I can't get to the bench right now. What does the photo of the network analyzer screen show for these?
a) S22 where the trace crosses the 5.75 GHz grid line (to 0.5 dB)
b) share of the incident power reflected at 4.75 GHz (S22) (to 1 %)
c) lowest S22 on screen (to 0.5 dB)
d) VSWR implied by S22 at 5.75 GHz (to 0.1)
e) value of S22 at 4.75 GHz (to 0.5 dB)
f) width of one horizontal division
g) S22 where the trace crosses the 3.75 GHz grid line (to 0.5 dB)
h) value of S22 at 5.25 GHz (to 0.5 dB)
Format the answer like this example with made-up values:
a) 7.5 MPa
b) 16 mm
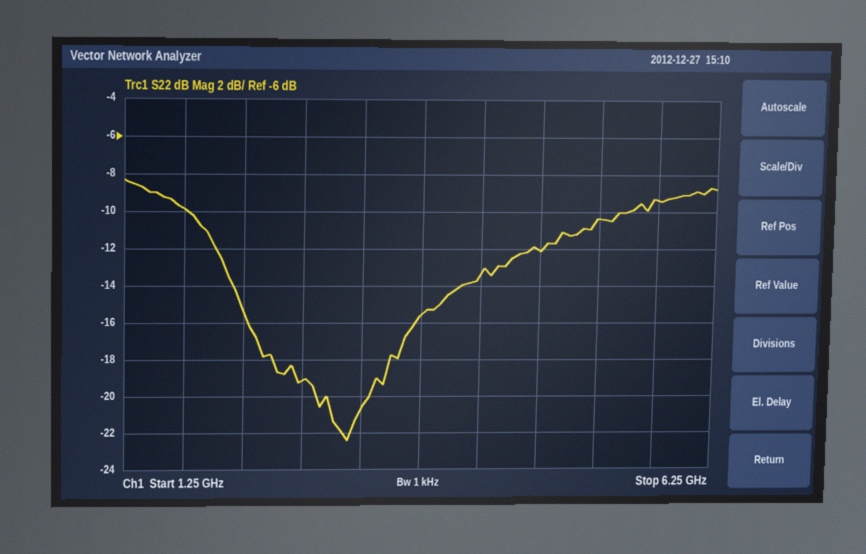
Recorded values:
a) -9.5 dB
b) 6 %
c) -22.5 dB
d) 2.0
e) -12.0 dB
f) 500 MHz
g) -15.5 dB
h) -10.5 dB
